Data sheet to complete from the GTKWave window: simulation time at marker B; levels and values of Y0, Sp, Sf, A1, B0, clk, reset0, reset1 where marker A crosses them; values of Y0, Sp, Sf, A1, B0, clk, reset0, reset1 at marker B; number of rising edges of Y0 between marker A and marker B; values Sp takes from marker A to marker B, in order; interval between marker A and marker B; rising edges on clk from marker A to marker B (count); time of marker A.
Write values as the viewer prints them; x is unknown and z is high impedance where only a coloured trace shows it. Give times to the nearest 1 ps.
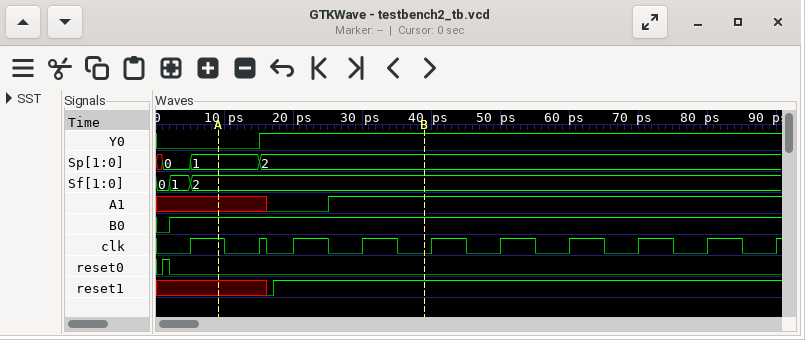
39 ps
Y0=0, Sp=1, Sf=2, A1=x, B0=1, clk=1, reset0=0, reset1=x
Y0=1, Sp=2, Sf=2, A1=1, B0=1, clk=0, reset0=0, reset1=1
1
1, 2
30 ps
3
9 ps
